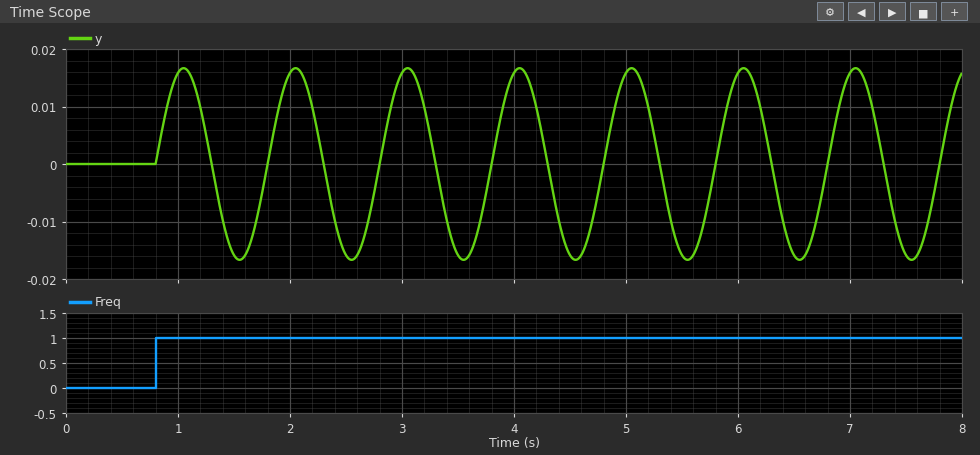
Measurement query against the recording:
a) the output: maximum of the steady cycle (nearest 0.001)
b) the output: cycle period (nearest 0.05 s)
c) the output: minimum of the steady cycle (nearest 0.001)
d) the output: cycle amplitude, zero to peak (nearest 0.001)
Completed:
0.017
1.00 s
-0.017
0.017
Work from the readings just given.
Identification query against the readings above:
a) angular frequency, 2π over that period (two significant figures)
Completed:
6.3 rad/s
